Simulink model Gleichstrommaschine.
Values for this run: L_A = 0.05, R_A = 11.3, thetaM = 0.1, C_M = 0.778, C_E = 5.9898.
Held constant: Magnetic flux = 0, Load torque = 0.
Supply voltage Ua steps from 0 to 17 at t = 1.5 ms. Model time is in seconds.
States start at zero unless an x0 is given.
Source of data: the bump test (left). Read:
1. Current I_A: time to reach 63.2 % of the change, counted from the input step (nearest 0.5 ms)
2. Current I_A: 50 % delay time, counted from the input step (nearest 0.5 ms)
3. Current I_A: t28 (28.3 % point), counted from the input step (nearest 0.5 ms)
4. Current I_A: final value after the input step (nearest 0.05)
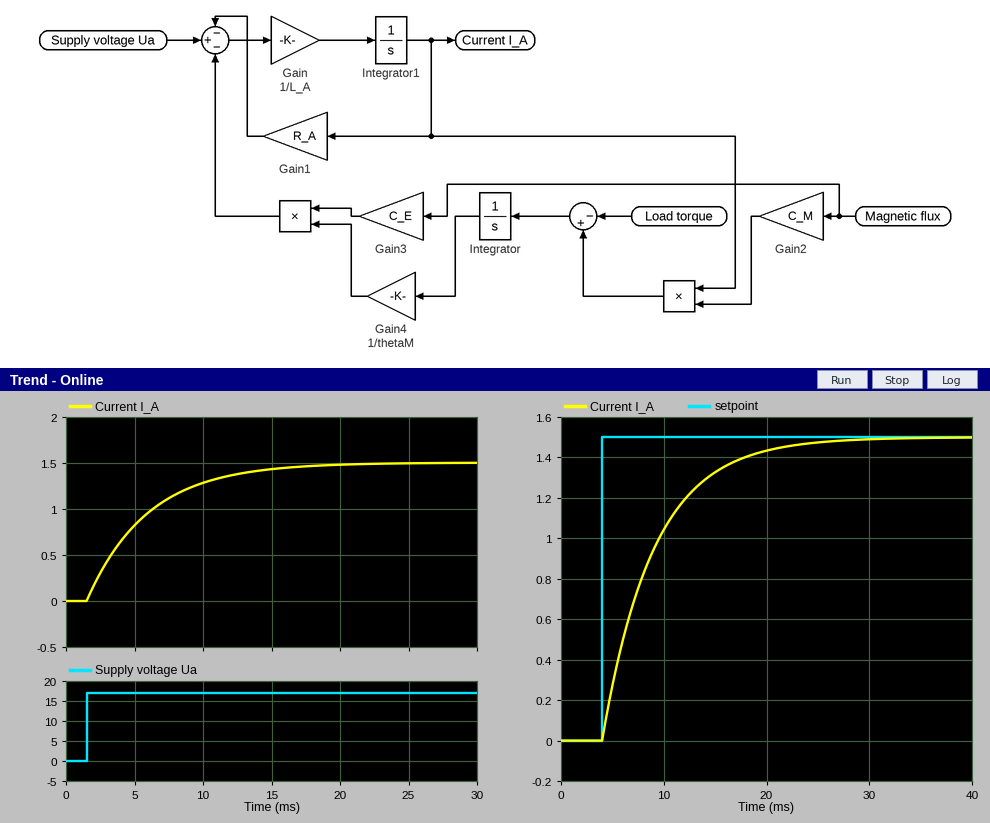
4.5 ms
3.0 ms
1.5 ms
1.50
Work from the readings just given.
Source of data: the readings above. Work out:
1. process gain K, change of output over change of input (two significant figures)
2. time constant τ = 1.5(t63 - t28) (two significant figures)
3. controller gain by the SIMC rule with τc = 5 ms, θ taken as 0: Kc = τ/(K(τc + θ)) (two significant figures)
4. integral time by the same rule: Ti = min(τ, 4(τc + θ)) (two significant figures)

0.088
4.5 ms
10
4.5 ms
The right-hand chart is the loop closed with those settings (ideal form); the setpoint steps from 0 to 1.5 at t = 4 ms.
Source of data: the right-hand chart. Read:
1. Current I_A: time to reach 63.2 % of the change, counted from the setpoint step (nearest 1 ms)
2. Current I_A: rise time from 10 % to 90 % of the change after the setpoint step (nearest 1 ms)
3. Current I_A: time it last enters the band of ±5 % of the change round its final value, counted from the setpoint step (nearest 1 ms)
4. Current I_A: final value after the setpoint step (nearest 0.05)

5 ms
11 ms
15 ms
1.50
